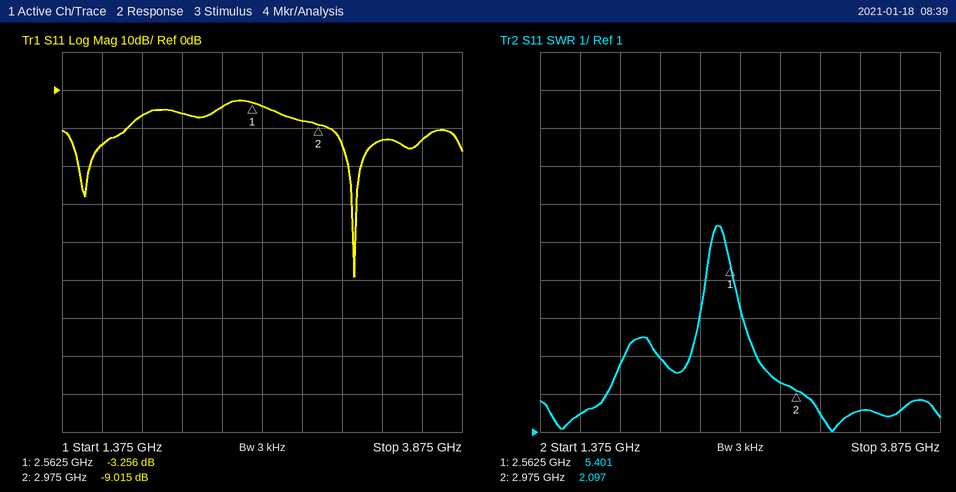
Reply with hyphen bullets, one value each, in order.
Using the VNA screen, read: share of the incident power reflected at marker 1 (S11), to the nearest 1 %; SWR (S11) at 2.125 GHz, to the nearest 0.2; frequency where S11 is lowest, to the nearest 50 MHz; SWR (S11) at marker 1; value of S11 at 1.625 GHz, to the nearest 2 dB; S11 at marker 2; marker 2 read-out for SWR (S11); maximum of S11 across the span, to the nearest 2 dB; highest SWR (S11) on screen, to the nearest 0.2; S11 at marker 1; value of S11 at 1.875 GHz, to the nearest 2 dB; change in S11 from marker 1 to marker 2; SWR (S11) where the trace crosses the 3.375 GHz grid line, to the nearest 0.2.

- 47 %
- 3.0
- 3.20 GHz
- 5.401
- -14 dB
- -9.015 dB
- 2.097
- -2 dB
- 6.4
- -3.256 dB
- -6 dB
- -5.759 dB
- 1.6
